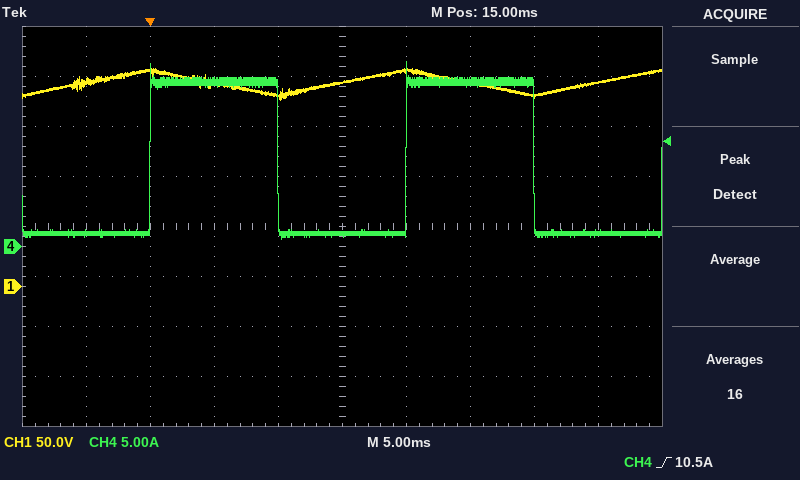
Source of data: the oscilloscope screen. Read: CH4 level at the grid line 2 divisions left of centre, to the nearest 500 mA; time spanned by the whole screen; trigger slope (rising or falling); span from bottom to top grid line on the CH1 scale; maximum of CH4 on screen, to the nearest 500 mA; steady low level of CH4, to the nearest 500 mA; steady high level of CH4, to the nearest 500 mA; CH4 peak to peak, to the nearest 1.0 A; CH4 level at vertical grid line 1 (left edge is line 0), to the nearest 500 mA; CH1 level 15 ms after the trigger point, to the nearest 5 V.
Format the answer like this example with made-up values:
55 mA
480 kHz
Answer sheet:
16.5 A
50 ms
rising
400 V
18.5 A
1.5 A
16.5 A
18.0 A
1.5 A
205 V
